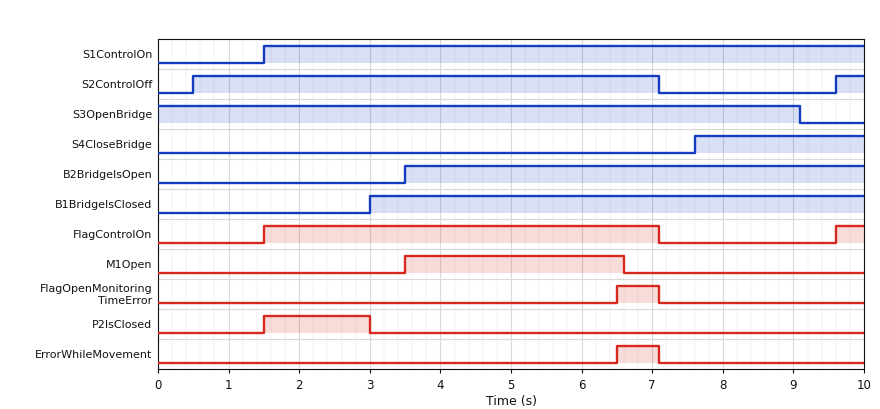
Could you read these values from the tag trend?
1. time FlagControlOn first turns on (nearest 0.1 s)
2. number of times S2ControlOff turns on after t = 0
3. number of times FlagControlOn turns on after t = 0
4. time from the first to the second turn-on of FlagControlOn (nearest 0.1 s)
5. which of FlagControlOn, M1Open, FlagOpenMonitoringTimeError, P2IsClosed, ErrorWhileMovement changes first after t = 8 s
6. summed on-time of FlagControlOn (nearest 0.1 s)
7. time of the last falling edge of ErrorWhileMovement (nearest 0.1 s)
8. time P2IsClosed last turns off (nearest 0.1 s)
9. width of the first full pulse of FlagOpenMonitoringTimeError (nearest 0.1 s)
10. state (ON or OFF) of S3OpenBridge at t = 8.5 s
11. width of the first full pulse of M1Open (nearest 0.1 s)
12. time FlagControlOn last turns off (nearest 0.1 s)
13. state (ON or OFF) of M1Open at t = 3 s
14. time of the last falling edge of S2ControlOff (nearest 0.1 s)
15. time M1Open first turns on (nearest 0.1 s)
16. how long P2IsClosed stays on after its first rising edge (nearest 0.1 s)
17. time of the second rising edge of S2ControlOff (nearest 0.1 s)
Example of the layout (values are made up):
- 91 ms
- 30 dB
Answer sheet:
- 1.5 s
- 2
- 2
- 8.1 s
- FlagControlOn
- 6.0 s
- 7.1 s
- 3.0 s
- 0.6 s
- ON
- 3.1 s
- 7.1 s
- OFF
- 7.1 s
- 3.5 s
- 1.5 s
- 9.6 s
